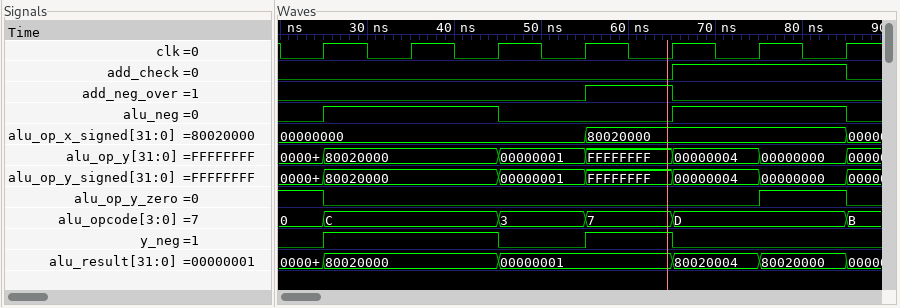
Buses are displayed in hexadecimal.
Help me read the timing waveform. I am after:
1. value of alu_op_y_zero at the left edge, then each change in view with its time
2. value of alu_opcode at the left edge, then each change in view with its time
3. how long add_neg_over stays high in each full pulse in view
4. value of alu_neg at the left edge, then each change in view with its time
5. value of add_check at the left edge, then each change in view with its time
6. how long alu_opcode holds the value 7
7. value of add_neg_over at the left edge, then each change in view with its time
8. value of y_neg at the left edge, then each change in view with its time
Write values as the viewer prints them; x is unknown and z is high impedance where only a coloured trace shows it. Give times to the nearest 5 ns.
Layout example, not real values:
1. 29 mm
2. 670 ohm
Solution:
1. 1, 0 at 25 ns, 1 at 75 ns, 0 at 85 ns
2. 0, C at 25 ns, 3 at 45 ns, 7 at 55 ns, D at 65 ns, B at 85 ns
3. 10 ns
4. 0, 1 at 25 ns, 0 at 45 ns, 1 at 65 ns, 0 at 85 ns
5. 0, 1 at 65 ns, 0 at 85 ns
6. 10 ns
7. 0, 1 at 55 ns, 0 at 65 ns
8. 0, 1 at 25 ns, 0 at 45 ns, 1 at 55 ns, 0 at 65 ns
